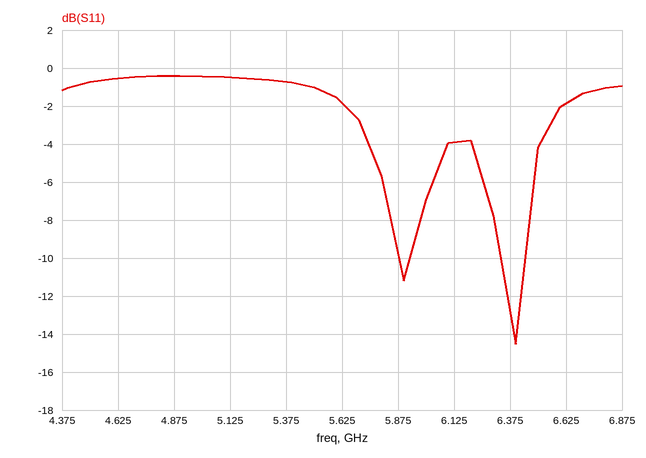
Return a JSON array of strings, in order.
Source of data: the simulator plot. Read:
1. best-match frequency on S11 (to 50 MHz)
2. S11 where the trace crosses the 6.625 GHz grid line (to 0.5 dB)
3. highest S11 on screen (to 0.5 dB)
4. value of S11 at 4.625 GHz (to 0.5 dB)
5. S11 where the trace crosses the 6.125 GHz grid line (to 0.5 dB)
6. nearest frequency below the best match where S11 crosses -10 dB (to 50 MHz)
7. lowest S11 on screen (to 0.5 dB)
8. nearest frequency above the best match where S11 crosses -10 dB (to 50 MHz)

["6.40 GHz", "-2.0 dB", "-0.5 dB", "-0.5 dB", "-4.0 dB", "6.35 GHz", "-14.5 dB", "6.45 GHz"]
